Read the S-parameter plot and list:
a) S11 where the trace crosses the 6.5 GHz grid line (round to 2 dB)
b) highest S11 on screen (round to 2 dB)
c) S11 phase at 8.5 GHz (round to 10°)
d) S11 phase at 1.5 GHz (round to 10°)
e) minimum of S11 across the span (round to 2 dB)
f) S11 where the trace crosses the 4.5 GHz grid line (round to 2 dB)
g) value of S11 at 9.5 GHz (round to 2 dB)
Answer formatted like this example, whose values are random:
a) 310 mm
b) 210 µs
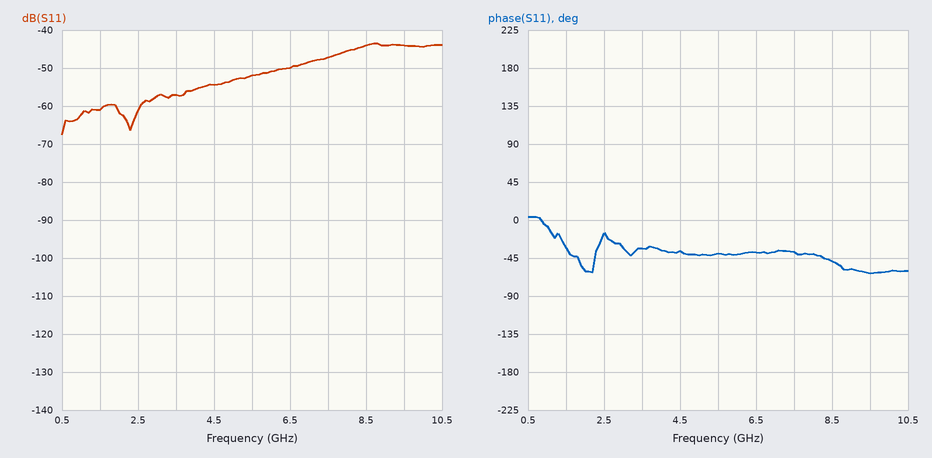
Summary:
a) -50 dB
b) -44 dB
c) -50°
d) -30°
e) -68 dB
f) -54 dB
g) -44 dB
